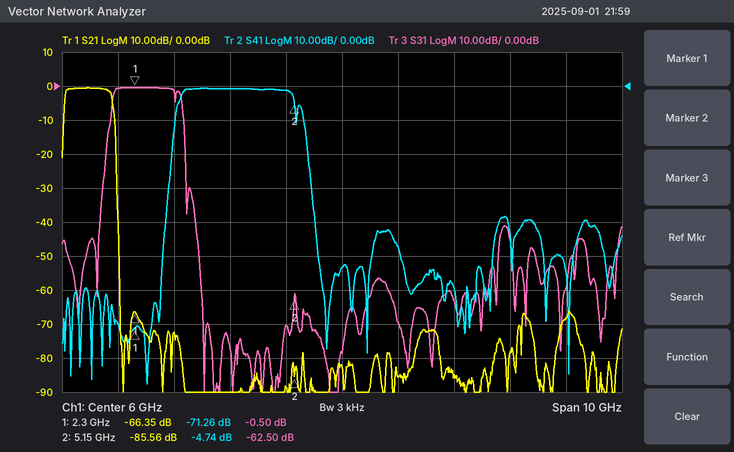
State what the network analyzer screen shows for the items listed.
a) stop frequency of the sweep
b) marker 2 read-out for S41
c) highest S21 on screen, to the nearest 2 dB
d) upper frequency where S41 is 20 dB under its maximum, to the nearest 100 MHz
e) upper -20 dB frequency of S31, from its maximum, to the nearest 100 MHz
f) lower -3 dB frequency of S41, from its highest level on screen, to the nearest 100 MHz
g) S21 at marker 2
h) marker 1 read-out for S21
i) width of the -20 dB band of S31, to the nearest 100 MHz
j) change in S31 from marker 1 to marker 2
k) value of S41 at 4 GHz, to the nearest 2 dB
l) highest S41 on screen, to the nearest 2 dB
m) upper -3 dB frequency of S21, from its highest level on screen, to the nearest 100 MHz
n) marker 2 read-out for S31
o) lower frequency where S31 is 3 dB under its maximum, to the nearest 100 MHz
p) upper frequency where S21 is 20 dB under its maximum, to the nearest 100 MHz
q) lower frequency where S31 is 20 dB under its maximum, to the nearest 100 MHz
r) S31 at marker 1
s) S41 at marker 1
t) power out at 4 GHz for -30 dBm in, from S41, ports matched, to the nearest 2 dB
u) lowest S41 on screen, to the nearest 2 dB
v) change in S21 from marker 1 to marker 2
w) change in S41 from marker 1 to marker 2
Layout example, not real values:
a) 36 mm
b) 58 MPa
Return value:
a) 11 GHz
b) -4.74 dB
c) 0 dB
d) 5.4 GHz
e) 3.2 GHz
f) 3.1 GHz
g) -85.56 dB
h) -66.35 dB
i) 1.4 GHz
j) -62.00 dB
k) 0 dB
l) 0 dB
m) 1.9 GHz
n) -62.50 dB
o) 1.9 GHz
p) 2.0 GHz
q) 1.8 GHz
r) -0.50 dB
s) -71.26 dB
t) -30 dBm
u) -88 dB
v) -19.21 dB
w) 66.52 dB
